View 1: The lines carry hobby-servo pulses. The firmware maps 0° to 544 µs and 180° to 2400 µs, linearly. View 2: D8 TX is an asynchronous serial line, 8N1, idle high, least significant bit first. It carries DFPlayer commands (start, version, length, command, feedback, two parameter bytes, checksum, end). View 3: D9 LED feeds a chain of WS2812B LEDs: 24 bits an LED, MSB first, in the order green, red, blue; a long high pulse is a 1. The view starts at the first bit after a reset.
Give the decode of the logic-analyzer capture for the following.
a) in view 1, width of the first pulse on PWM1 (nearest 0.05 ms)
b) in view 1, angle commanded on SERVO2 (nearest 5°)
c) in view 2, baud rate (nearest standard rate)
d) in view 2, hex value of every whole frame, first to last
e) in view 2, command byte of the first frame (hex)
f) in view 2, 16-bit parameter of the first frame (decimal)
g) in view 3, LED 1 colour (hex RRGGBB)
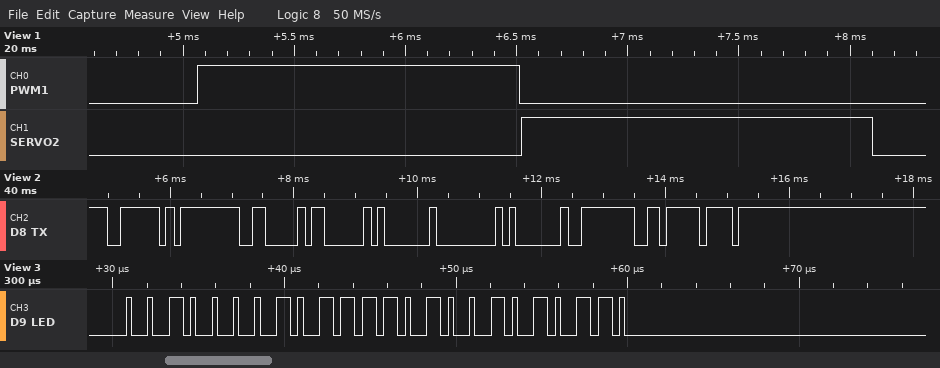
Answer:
1.45 ms
100°
9600 baud
7E FF 06 03 01 00 01 FE F6 EF
0x03
1
#7A2156
